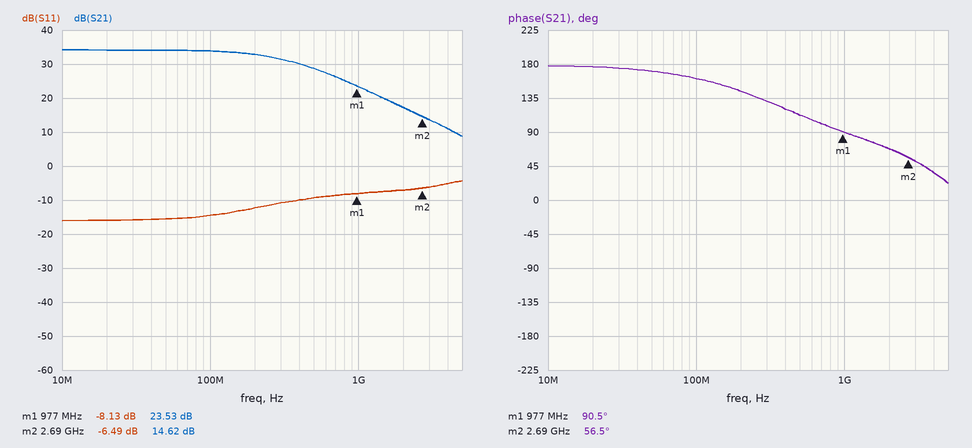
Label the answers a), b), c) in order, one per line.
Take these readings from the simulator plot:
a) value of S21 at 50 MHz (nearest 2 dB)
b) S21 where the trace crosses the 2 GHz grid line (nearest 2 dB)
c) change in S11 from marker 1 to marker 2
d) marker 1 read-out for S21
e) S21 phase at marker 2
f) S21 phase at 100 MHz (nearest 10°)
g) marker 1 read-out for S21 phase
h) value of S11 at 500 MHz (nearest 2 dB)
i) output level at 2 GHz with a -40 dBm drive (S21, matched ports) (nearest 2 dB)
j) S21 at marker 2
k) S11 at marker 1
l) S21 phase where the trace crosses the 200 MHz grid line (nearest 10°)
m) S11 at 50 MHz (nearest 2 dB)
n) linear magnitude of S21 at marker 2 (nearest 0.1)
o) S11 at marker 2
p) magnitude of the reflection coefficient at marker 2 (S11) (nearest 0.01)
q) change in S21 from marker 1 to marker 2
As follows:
a) 34 dB
b) 18 dB
c) 1.64 dB
d) 23.53 dB
e) 56.5°
f) 160°
g) 90.5°
h) -10 dB
i) -22 dBm
j) 14.62 dB
k) -8.13 dB
l) 140°
m) -16 dB
n) 5.4
o) -6.49 dB
p) 0.47
q) -8.91 dB
